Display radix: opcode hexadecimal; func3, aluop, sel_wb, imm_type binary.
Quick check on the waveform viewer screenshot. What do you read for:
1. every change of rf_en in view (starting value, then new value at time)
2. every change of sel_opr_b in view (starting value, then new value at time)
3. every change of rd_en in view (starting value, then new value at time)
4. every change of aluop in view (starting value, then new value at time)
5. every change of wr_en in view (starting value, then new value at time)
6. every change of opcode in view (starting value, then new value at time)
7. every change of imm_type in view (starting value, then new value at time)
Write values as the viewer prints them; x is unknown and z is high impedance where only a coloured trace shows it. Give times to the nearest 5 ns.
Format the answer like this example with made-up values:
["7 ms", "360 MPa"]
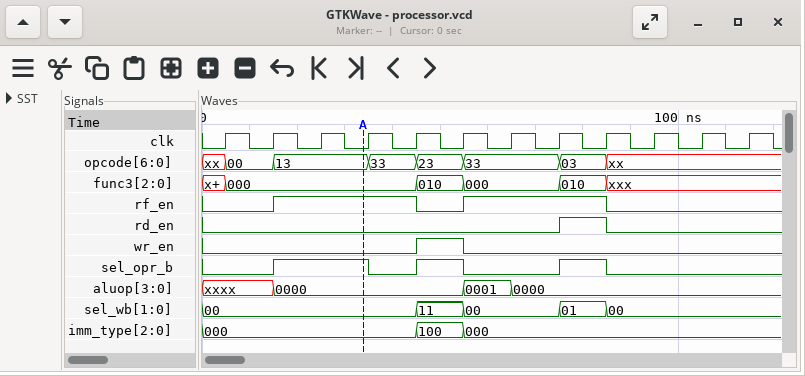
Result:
["0, 1 at 15 ns, 0 at 45 ns, 1 at 55 ns, 0 at 85 ns", "0, 1 at 15 ns, 0 at 35 ns, 1 at 45 ns, 0 at 55 ns, 1 at 75 ns, 0 at 85 ns", "0, 1 at 75 ns, 0 at 85 ns", "xxxx, 0000 at 15 ns, 0001 at 55 ns, 0000 at 65 ns", "0, 1 at 45 ns, 0 at 55 ns", "xx, 00 at 5 ns, 13 at 15 ns, 33 at 35 ns, 23 at 45 ns, 33 at 55 ns, 03 at 75 ns, xx at 85 ns", "000, 100 at 45 ns, 000 at 55 ns"]
